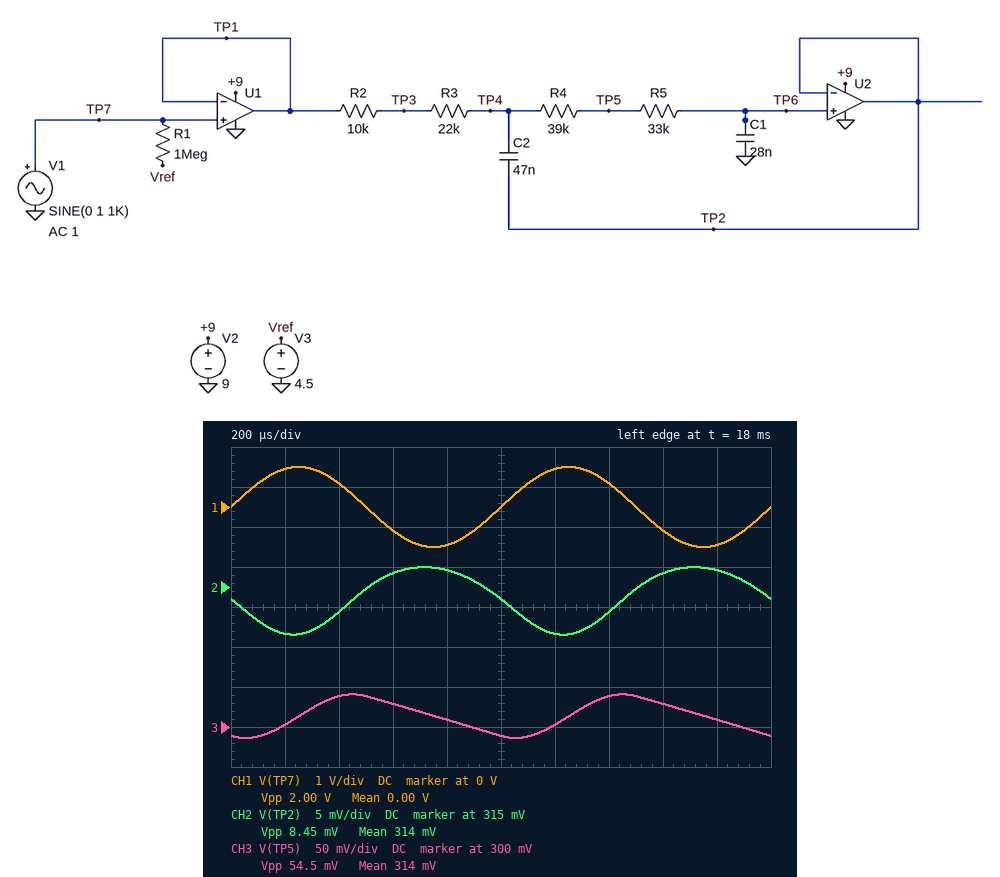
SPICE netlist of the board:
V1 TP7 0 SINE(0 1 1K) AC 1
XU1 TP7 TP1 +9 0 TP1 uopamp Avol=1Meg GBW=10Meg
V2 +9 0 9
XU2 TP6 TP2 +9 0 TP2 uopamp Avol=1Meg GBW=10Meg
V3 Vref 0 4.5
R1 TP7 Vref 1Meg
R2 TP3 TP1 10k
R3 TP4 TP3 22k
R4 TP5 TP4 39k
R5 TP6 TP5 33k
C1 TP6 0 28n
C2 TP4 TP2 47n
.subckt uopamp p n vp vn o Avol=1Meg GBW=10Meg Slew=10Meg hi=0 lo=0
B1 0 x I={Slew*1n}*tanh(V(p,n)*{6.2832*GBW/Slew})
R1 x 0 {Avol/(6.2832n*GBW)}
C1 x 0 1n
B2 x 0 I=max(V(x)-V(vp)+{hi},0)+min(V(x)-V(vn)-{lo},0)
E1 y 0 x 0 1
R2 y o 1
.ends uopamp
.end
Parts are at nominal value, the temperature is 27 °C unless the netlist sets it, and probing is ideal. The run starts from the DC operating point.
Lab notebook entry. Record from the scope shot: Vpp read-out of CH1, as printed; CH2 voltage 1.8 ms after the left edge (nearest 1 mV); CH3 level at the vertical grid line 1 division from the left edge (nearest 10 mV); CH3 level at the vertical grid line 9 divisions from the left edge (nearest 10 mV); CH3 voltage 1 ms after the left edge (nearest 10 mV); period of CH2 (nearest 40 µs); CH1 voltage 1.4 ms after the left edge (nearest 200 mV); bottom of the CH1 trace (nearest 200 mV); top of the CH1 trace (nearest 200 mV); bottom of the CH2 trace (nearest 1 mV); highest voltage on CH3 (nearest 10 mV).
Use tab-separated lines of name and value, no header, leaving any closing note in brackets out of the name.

Vpp read-out of CH1, as printed	2.00 V
CH2 voltage 1.8 ms after the left edge	317 mV
CH3 level at the vertical grid line 1 division from the left edge	300 mV
CH3 level at the vertical grid line 9 divisions from the left edge	310 mV
CH3 voltage 1 ms after the left edge	290 mV
period of CH2	1.00 ms
CH1 voltage 1.4 ms after the left edge	600 mV
bottom of the CH1 trace	-1.0 V
top of the CH1 trace	1.0 V
bottom of the CH2 trace	309 mV
highest voltage on CH3	340 mV
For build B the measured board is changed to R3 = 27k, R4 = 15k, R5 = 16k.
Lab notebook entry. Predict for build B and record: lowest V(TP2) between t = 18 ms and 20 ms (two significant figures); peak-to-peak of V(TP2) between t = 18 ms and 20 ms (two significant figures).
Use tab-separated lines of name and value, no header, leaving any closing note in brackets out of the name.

lowest V(TP2) between t = 18 ms and 20 ms	300 mV
peak-to-peak of V(TP2) between t = 18 ms and 20 ms	17 mV
